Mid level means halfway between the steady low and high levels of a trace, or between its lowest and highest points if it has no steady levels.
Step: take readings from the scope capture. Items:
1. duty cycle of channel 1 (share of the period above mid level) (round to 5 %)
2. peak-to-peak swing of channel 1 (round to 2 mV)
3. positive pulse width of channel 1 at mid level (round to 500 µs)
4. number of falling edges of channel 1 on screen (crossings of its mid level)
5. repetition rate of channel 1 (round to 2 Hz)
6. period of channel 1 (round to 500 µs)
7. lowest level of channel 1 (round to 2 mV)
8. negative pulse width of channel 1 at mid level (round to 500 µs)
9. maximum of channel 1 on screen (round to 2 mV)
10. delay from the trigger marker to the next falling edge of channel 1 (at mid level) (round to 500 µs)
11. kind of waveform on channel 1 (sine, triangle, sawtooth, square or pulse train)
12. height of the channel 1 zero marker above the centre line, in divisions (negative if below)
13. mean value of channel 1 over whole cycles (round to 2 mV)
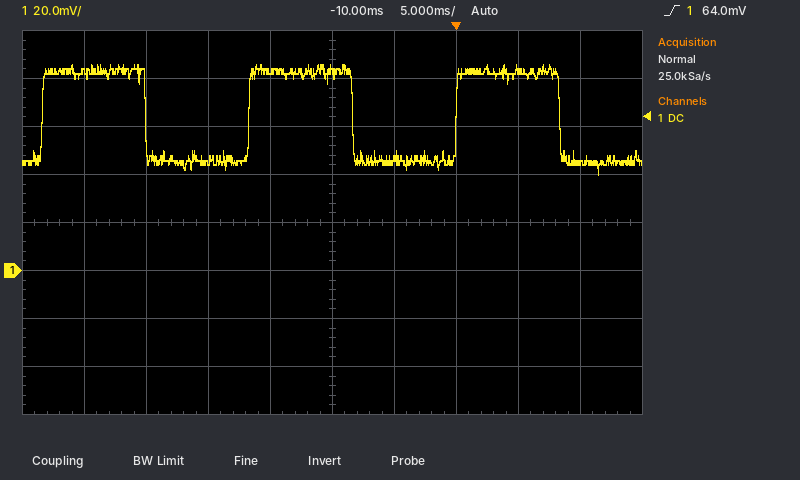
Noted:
50 %
46 mV
8.5 ms
3
60 Hz
16.5 ms
40 mV
8.5 ms
86 mV
8.5 ms
square
-1.0 div
64 mV
